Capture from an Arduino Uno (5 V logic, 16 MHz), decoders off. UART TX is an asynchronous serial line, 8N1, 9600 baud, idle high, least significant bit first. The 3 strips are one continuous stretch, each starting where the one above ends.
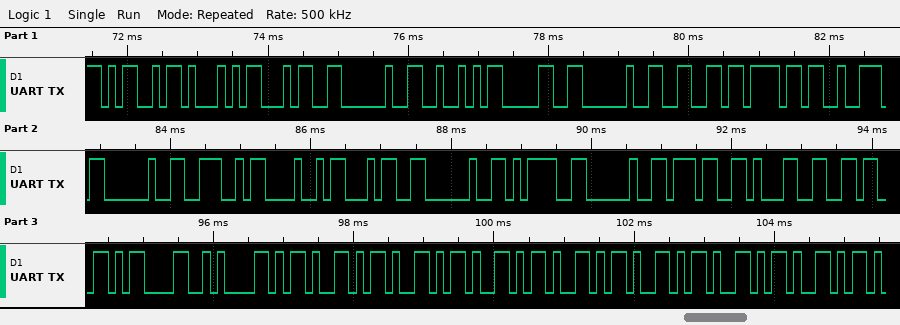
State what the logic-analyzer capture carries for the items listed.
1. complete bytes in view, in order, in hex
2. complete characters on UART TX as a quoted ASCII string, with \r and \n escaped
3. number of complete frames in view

4D 51 34 20 52 30 20 66 6F 72 20 4E 48 34 20 3D 20 37 31 36 0D 0A 2D 2D 2D 2D 2D 2D 2D
"MQ4 R0 for NH4 = 716\r\n-------"
29
